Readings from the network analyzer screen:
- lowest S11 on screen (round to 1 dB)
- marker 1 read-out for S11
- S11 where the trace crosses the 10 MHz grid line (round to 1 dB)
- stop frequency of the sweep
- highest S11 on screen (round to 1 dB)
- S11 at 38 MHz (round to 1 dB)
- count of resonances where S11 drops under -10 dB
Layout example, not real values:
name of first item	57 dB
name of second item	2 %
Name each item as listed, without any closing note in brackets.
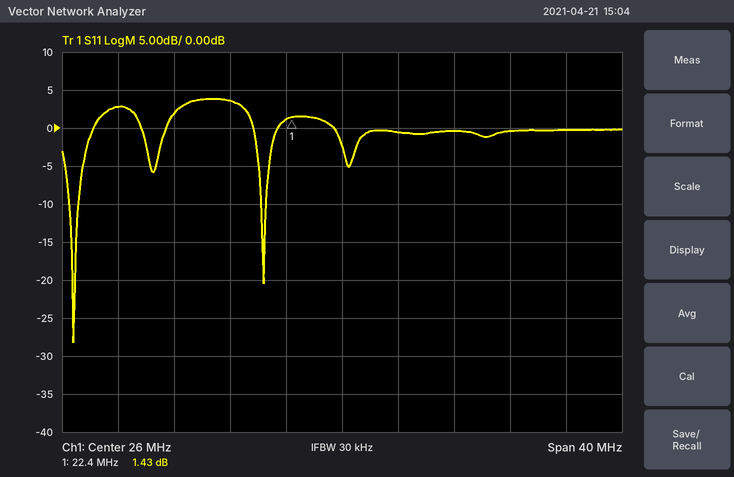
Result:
lowest S11 on screen	-28 dB
marker 1 read-out for S11	1.43 dB
S11 where the trace crosses the 10 MHz grid line	3 dB
stop frequency of the sweep	46 MHz
highest S11 on screen	4 dB
S11 at 38 MHz	0 dB
count of resonances where S11 drops under -10 dB	2
